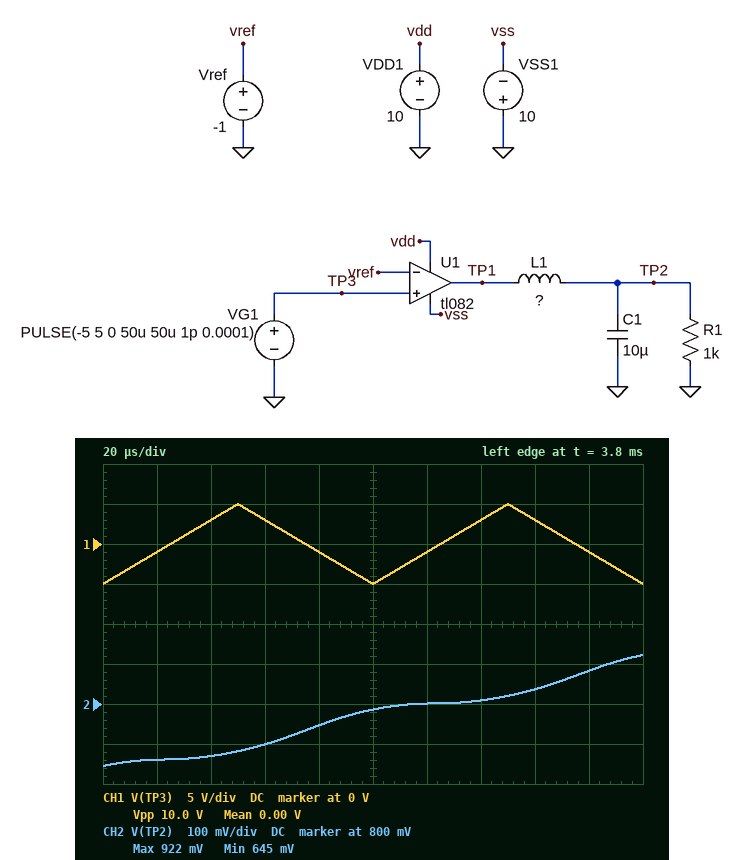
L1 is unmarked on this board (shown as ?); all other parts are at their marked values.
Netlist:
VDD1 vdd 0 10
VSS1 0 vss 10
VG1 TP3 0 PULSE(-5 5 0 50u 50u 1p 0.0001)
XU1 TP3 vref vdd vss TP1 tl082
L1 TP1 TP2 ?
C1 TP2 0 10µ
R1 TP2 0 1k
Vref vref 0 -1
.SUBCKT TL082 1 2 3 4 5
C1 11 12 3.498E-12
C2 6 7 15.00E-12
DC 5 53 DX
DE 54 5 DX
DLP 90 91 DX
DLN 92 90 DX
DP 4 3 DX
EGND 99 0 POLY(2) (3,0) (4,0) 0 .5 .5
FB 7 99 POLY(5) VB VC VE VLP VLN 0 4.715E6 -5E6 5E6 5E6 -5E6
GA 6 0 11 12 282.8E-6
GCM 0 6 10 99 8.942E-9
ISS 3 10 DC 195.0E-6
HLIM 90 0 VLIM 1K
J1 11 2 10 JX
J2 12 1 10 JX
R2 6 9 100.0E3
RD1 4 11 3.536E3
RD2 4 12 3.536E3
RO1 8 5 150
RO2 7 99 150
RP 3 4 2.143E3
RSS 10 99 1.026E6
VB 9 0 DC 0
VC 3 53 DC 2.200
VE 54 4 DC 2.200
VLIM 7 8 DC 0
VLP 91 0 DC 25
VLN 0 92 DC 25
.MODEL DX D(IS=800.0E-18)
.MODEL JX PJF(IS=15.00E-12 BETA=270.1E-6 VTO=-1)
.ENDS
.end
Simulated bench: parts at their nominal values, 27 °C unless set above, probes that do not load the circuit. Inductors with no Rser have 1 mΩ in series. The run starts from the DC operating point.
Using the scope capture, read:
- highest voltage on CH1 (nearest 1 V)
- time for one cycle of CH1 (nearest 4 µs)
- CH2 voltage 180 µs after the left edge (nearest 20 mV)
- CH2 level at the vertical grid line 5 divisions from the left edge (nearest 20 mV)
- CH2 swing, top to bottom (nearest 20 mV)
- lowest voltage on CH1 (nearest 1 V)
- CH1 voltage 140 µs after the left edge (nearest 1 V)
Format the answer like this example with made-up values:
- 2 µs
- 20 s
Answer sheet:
- 5 V
- 100 µs
- 880 mV
- 780 mV
- 280 mV
- -5 V
- 3 V
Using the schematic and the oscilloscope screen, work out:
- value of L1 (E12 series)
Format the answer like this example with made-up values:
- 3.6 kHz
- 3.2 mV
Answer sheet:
- 15 mH
